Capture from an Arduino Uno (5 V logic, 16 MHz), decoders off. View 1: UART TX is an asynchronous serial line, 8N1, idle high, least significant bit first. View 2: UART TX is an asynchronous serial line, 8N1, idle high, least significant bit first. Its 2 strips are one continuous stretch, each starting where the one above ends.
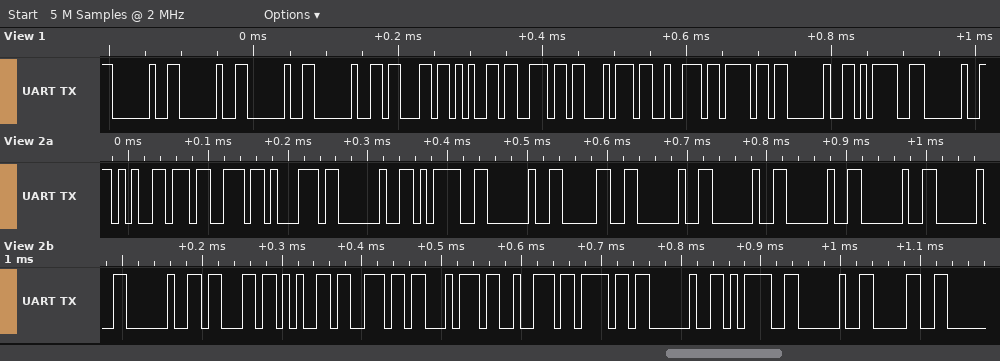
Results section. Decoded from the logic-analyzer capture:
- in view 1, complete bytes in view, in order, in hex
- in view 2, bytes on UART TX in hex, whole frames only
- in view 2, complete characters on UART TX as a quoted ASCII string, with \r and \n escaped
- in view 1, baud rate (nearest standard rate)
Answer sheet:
20 20 20 20 63 65 6E 74 72 6F 20 3D 20
65 73 71 20 3D 20 30 20 20 20 20 20 20 63 65 6E 74 72 6F 20 3D 20 30
"esq = 0      centro = 0"
115200 baud
